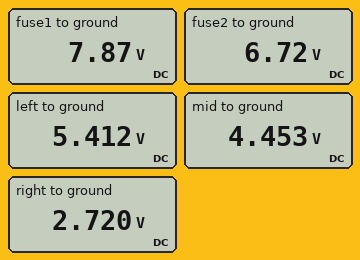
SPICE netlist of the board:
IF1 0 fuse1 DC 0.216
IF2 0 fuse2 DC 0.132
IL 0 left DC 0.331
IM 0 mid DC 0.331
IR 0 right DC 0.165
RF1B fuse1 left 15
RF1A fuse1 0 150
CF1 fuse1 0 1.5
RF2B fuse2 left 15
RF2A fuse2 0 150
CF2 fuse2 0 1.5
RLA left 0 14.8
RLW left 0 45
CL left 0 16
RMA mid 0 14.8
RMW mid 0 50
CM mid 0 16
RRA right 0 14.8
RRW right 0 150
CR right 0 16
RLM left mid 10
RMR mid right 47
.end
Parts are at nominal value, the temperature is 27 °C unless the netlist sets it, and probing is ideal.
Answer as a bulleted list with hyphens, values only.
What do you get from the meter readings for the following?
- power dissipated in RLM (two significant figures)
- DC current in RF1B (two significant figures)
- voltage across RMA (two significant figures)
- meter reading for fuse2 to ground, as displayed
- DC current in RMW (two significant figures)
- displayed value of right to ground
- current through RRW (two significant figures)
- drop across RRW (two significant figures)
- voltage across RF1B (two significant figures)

- 92 mW
- 160 mA
- 4.5 V
- 6.72 V
- 89 mA
- 2.720 V
- 18 mA
- 2.7 V
- 2.5 V
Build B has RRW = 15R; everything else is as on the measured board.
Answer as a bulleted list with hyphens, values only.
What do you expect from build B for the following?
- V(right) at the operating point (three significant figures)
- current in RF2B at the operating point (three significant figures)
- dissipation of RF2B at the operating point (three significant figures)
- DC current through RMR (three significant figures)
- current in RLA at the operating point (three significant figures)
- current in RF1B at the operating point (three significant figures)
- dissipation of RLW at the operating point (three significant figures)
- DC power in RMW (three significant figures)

- 1.65 V
- 87.6 mA
- 115 mW
- 56.6 mA
- 361 mA
- 164 mA
- 634 mW
- 372 mW
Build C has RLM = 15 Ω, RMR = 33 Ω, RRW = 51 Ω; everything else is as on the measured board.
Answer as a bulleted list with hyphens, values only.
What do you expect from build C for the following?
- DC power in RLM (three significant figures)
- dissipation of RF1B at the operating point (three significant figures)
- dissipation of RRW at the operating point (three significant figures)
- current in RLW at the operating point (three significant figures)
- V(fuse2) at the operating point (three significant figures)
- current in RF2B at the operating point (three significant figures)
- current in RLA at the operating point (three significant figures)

- 114 mW
- 399 mW
- 121 mW
- 122 mA
- 6.80 V
- 86.7 mA
- 371 mA
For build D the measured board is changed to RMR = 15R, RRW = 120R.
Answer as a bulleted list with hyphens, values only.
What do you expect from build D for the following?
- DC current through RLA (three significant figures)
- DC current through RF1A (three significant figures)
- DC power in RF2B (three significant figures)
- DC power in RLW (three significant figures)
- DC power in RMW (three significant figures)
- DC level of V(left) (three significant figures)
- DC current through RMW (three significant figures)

- 357 mA
- 51.7 mA
- 116 mW
- 621 mW
- 353 mW
- 5.29 V
- 84.0 mA
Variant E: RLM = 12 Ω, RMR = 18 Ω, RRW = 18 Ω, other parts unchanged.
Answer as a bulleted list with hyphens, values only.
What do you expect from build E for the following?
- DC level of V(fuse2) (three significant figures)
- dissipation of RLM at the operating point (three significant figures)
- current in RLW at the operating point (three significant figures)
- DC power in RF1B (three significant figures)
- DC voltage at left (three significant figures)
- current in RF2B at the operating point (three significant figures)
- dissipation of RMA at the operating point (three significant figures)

- 6.58 V
- 149 mW
- 117 mA
- 406 mW
- 5.26 V
- 88.1 mA
- 1.04 W
